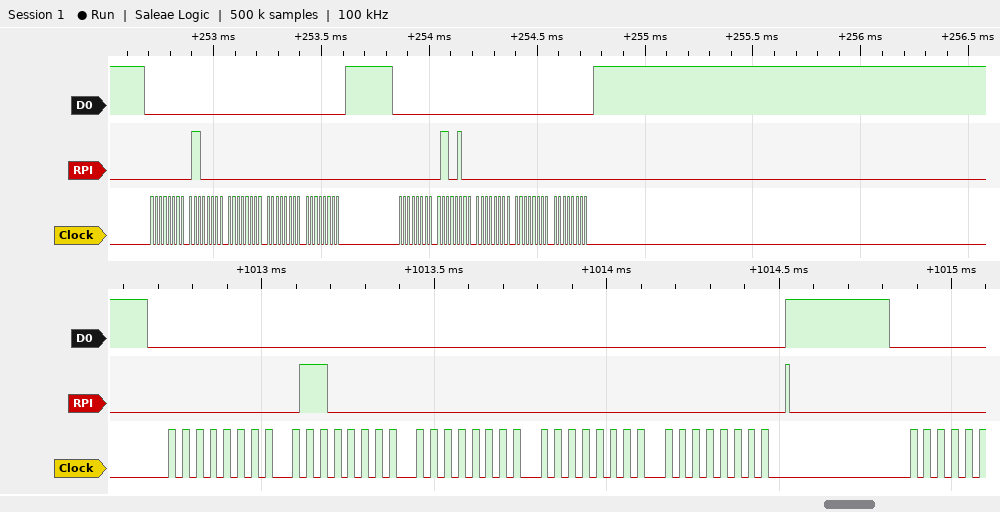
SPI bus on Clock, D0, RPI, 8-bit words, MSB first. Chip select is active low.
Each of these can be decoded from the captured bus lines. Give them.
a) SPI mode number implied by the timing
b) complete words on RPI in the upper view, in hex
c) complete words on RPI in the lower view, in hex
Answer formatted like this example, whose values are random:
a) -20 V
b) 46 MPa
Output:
a) 0
b) 00, 60, 00, 00, 00, 00, 64, 00, 00, 00
c) 00, 60, 00, 00, 00
